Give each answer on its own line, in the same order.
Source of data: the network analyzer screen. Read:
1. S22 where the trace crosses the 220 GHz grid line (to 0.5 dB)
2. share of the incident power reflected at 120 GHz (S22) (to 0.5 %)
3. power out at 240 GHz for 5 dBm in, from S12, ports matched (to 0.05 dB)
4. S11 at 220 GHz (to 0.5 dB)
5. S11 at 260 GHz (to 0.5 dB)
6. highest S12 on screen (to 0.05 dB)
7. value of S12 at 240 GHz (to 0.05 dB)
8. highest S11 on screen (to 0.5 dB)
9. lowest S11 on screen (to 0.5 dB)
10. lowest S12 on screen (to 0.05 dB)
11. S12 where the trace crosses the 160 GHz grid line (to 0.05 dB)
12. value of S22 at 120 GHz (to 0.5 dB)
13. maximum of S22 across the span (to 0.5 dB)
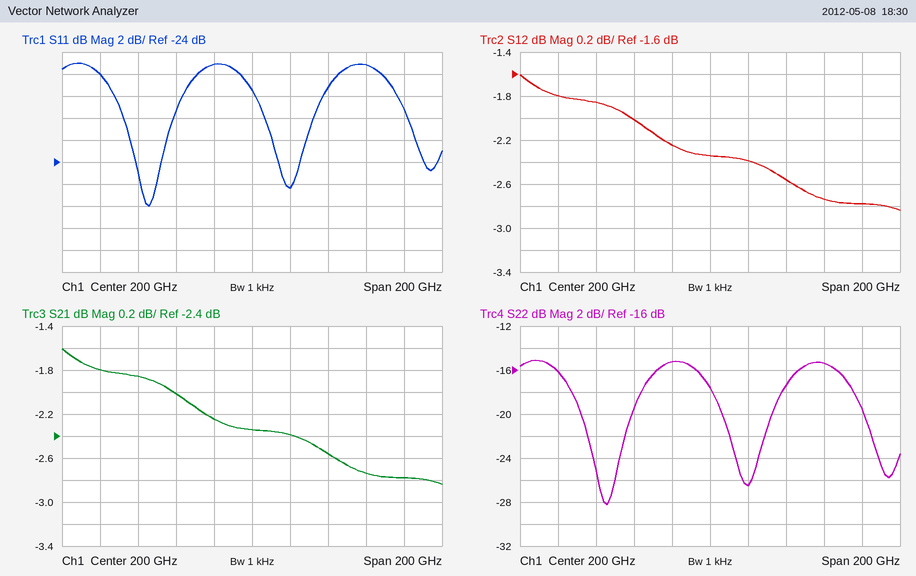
-26.5 dB
2.5 %
2.45 dBm
-26.5 dB
-15.0 dB
-1.60 dB
-2.55 dB
-15.0 dB
-28.0 dB
-2.85 dB
-2.00 dB
-16.0 dB
-15.0 dB
